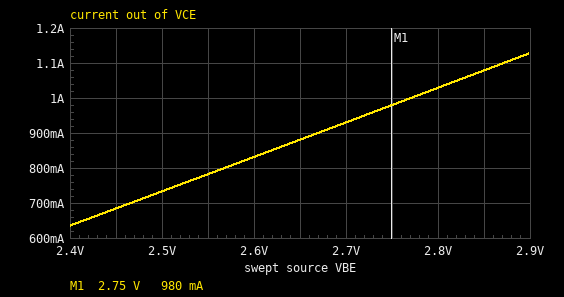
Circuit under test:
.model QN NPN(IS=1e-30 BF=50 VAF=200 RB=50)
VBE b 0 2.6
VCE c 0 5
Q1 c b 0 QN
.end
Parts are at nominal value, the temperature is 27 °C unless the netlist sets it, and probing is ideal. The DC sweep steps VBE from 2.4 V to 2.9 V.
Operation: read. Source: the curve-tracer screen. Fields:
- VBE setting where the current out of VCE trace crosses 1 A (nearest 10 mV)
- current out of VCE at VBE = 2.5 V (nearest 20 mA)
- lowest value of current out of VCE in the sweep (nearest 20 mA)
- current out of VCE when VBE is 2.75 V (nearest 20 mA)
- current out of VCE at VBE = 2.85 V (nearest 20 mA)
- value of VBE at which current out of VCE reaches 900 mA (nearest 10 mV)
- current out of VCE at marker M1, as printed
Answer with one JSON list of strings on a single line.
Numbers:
["2.77 V", "740 mA", "640 mA", "980 mA", "1.08 A", "2.67 V", "980 mA"]
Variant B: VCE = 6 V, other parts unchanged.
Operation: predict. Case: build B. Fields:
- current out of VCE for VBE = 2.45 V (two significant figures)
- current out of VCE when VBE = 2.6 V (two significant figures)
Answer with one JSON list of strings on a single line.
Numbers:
["690 mA", "840 mA"]
